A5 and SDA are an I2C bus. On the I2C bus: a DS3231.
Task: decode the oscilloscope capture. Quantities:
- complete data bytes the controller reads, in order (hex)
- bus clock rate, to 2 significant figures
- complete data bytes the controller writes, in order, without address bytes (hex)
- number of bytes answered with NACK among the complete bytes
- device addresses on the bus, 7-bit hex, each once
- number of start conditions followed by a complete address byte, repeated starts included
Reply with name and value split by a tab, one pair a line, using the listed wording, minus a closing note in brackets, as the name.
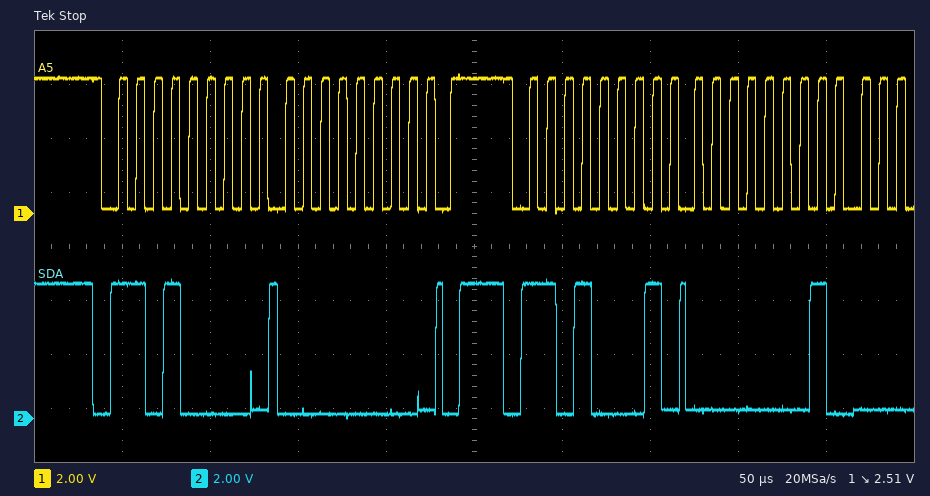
complete data bytes the controller reads, in order	01
bus clock rate, to 2 significant figures	100 kHz
complete data bytes the controller writes, in order, without address bytes	00
number of bytes answered with NACK among the complete bytes	0
device addresses on the bus, 7-bit hex, each once	0x68
number of start conditions followed by a complete address byte, repeated starts included	2
